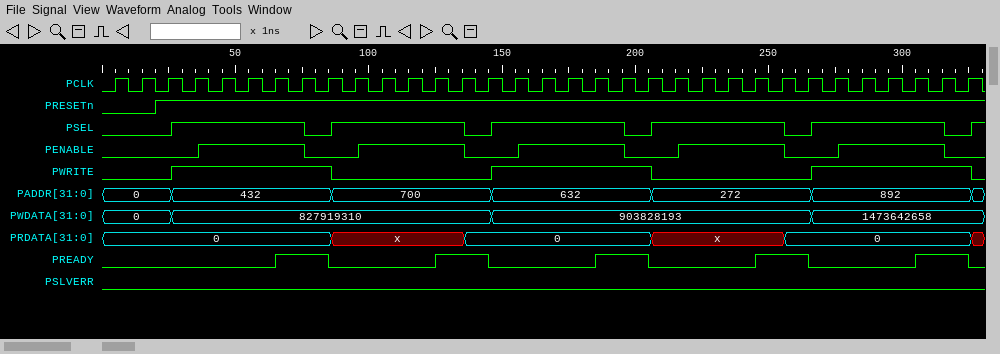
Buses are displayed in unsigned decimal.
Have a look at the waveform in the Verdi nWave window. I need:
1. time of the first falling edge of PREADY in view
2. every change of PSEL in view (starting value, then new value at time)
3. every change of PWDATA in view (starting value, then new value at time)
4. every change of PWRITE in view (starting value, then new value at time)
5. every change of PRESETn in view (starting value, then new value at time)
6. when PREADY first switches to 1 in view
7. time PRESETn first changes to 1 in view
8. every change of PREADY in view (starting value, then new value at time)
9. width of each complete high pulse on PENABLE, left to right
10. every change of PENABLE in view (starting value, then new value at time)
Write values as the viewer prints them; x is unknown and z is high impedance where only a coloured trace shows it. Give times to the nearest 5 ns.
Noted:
85 ns
0, 1 at 25 ns, 0 at 75 ns, 1 at 85 ns, 0 at 135 ns, 1 at 145 ns, 0 at 195 ns, 1 at 205 ns, 0 at 255 ns, 1 at 265 ns, 0 at 315 ns, 1 at 325 ns
0, 827919310 at 25 ns, 903828193 at 145 ns, 1473642658 at 265 ns
0, 1 at 25 ns, 0 at 85 ns, 1 at 145 ns, 0 at 205 ns, 1 at 265 ns, 0 at 325 ns
0, 1 at 20 ns
65 ns
20 ns
0, 1 at 65 ns, 0 at 85 ns, 1 at 125 ns, 0 at 145 ns, 1 at 185 ns, 0 at 205 ns, 1 at 245 ns, 0 at 265 ns, 1 at 305 ns, 0 at 325 ns
40 ns, 40 ns, 40 ns, 40 ns, 40 ns
0, 1 at 35 ns, 0 at 75 ns, 1 at 95 ns, 0 at 135 ns, 1 at 155 ns, 0 at 195 ns, 1 at 215 ns, 0 at 255 ns, 1 at 275 ns, 0 at 315 ns
